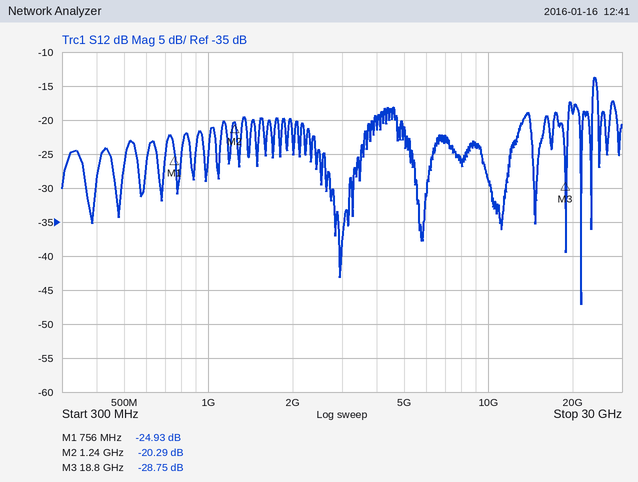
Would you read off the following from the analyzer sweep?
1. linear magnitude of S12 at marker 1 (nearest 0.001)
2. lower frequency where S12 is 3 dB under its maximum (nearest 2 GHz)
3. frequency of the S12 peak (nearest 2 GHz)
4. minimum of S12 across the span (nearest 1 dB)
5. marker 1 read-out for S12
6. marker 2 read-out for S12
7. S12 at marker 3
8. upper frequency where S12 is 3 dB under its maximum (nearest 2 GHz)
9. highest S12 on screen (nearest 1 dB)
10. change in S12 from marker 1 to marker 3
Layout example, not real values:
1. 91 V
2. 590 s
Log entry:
1. 0.057
2. 24 GHz
3. 24 GHz
4. -47 dB
5. -24.93 dB
6. -20.29 dB
7. -28.75 dB
8. 24 GHz
9. -14 dB
10. -3.82 dB
